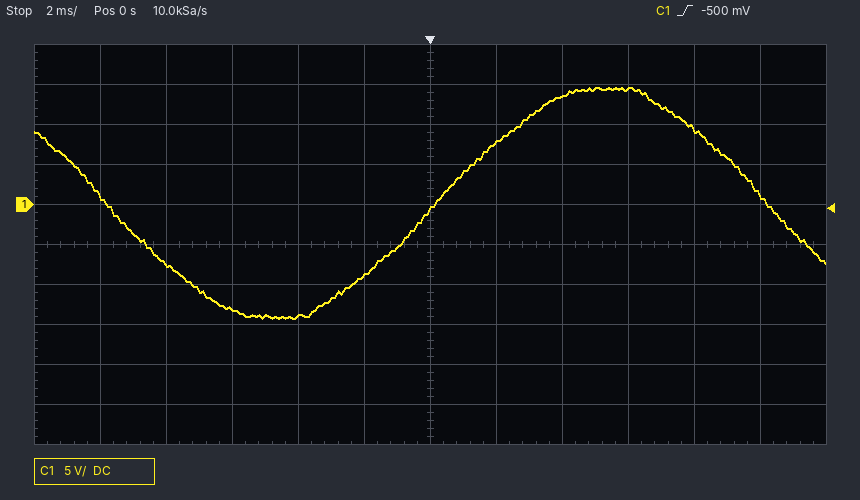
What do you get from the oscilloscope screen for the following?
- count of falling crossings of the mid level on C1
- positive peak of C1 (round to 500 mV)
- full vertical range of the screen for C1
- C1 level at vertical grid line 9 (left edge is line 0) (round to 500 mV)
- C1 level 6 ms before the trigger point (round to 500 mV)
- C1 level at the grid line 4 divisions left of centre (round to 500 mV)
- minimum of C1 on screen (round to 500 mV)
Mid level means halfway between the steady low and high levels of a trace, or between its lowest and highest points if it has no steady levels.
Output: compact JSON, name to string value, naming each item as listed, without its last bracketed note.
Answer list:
{"count of falling crossings of the mid level on C1": "2", "positive peak of C1": "14.5 V", "full vertical range of the screen for C1": "50 V", "C1 level at vertical grid line 9 (left edge is line 0)": "14.5 V", "C1 level 6 ms before the trigger point": "-13.0 V", "C1 level at the grid line 4 divisions left of centre": "-7.5 V", "minimum of C1 on screen": "-14.0 V"}
